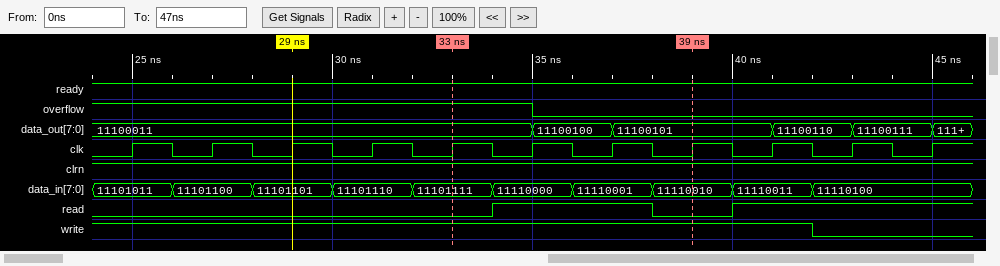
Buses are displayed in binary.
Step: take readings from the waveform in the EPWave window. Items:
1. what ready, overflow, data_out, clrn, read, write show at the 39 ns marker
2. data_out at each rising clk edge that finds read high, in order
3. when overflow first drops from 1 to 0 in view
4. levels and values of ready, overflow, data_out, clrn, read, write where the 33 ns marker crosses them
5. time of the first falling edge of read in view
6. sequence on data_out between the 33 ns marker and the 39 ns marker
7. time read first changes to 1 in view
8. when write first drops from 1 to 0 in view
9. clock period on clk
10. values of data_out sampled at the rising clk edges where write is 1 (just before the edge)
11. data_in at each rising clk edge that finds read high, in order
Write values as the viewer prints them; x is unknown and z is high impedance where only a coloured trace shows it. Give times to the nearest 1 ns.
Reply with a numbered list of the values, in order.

1. ready=1, overflow=0, data_out=11100101, clrn=1, read=0, write=1
2. 11100011, 11100100, 11100101, 11100110, 11100111
3. 35 ns
4. ready=1, overflow=1, data_out=11100011, clrn=1, read=0, write=1
5. 38 ns
6. 11100011, 11100100, 11100101
7. 34 ns
8. 42 ns
9. 2 ns
10. 11100011, 11100011, 11100011, 11100011, 11100011, 11100011, 11100100, 11100101, 11100101
11. 11110000, 11110001, 11110011, 11110100, 11110100
